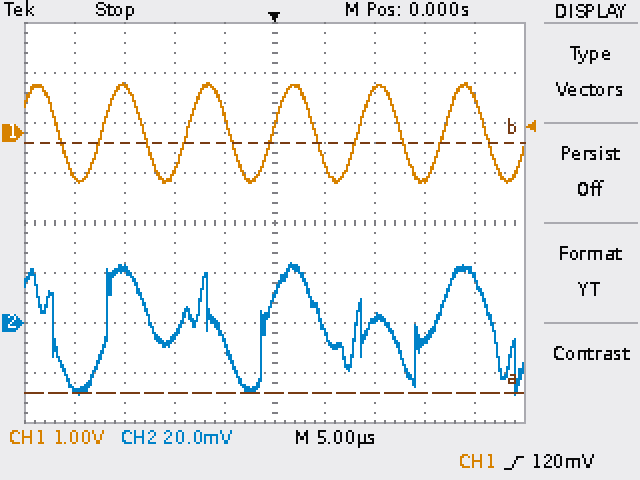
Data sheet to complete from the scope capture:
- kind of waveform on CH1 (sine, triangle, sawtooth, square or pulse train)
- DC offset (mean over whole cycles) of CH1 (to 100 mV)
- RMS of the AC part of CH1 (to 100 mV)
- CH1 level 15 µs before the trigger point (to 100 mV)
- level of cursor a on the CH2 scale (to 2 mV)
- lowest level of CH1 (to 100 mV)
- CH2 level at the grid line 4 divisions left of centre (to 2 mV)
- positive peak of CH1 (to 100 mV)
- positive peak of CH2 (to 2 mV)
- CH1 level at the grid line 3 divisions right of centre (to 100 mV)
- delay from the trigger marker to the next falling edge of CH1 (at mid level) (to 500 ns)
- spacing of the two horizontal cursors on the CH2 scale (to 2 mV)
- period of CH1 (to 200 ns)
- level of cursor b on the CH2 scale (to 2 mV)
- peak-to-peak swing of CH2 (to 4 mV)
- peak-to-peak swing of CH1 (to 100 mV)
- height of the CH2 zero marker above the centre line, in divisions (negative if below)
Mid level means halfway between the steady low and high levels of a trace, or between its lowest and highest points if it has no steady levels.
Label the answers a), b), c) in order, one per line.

a) sine
b) 0.0 V
c) 700 mV
d) 900 mV
e) -28 mV
f) -1.0 V
g) -26 mV
h) 1.0 V
i) 24 mV
j) -900 mV
k) 4.0 µs
l) 100 mV
m) 8.6 µs
n) 72 mV
o) 52 mV
p) 2.0 V
q) -2.0 div
